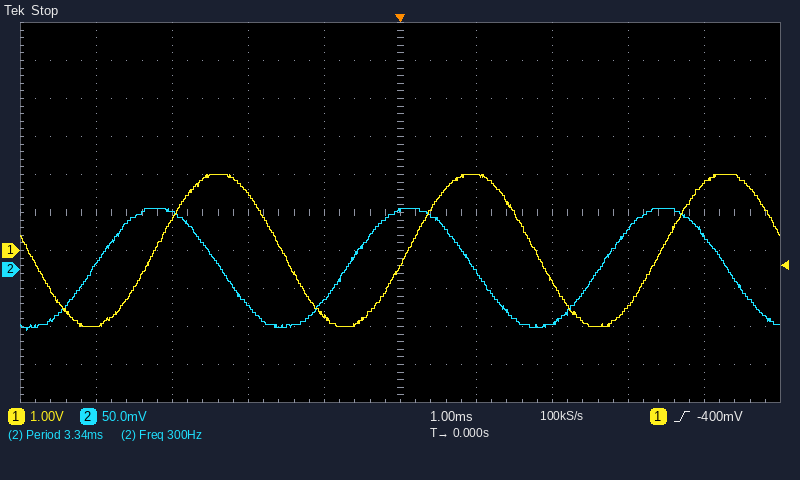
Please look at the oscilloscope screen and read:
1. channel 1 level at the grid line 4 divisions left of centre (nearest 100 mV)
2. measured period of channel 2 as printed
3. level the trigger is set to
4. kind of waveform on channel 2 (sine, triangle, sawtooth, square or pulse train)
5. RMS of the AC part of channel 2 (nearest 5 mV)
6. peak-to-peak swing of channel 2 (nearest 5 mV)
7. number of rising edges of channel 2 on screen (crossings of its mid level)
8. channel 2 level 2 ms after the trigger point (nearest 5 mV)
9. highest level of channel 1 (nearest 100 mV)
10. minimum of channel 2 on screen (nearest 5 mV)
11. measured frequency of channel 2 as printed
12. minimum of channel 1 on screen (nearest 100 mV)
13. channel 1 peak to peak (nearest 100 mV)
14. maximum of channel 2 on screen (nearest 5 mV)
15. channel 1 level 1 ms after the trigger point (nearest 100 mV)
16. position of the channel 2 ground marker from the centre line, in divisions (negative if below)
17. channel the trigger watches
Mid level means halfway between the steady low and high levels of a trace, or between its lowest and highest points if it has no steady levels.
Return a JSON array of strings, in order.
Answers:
["-2.0 V", "3.34 ms", "-400 mV", "sine", "55 mV", "160 mV", "3", "-70 mV", "2.0 V", "-80 mV", "300 Hz", "-2.0 V", "4.0 V", "80 mV", "2.0 V", "-1.5 div", "channel 1"]
